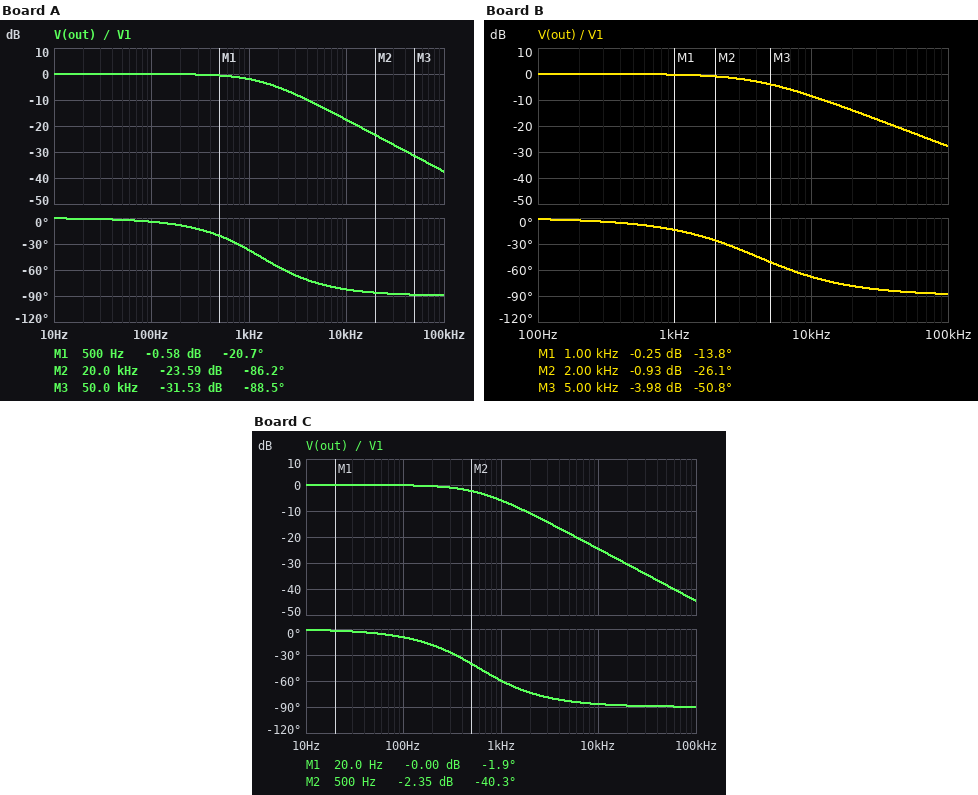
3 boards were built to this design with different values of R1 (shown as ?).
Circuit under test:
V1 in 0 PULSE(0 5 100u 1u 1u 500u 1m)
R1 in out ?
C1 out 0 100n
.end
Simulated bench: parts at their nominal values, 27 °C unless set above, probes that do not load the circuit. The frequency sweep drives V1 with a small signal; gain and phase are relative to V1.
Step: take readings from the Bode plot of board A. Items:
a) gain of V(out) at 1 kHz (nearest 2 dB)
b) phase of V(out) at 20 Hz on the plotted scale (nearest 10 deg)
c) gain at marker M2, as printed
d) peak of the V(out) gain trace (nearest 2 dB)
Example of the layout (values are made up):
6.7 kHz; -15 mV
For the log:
-2 dB; 0 deg; -23.59 dB; 0 dB
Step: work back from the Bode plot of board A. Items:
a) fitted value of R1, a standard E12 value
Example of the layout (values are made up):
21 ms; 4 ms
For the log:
1.2 kΩ
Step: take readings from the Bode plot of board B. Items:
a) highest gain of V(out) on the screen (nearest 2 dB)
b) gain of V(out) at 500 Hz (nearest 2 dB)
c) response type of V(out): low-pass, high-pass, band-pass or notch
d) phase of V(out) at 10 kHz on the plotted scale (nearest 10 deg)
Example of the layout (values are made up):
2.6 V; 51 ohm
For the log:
0 dB; 0 dB; low-pass; -70 deg
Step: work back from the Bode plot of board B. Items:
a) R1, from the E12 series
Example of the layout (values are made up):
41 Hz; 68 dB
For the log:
390 Ω
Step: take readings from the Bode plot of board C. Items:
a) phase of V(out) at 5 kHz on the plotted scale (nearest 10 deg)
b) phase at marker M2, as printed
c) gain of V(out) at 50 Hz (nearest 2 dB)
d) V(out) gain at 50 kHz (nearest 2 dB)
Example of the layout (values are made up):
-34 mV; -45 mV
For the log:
-80 deg; -40.3 deg; 0 dB; -38 dB
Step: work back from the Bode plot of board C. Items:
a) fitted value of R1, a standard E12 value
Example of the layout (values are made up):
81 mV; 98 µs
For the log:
2.7 kΩ
